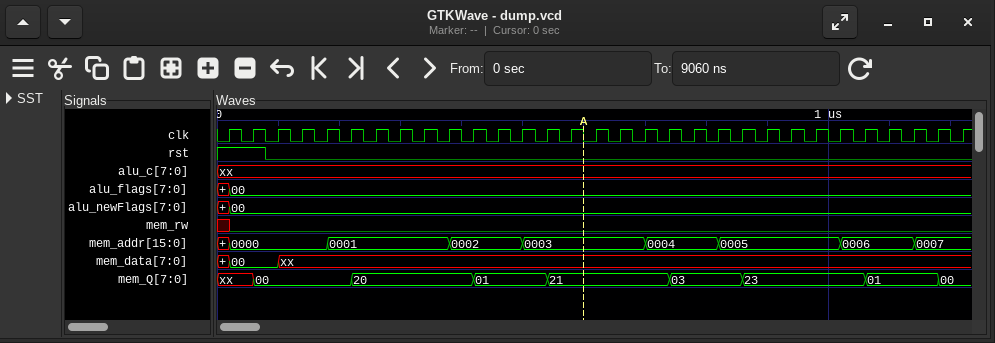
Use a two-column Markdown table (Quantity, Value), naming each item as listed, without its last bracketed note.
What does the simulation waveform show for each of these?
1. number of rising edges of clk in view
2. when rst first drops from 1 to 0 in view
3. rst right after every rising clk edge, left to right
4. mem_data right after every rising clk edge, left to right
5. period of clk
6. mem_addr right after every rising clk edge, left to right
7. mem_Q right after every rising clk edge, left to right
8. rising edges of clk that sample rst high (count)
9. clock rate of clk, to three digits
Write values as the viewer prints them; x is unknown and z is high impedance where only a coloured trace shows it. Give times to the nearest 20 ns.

| Quantity | Value |
|---|---|
| number of rising edges of clk in view | 31 |
| when rst first drops from 1 to 0 in view | 80 ns |
| rst right after every rising clk edge, left to right | 1 1 0 0 0 0 0 0 0 0 0 0 0 0 0 0 0 0 0 0 0 0 0 0 0 0 0 0 0 0 0 |
| mem_data right after every rising clk edge, left to right | 00, 00, xx, xx, xx, xx, xx, xx, xx, xx, xx, xx, xx, xx, xx, xx, xx, xx, xx, xx, xx, xx, xx, xx, xx, xx, xx, xx, xx, xx, xx |
| period of clk | 40 ns |
| mem_addr right after every rising clk edge, left to right | 0000, 0000, 0000, 0000, 0001, 0001, 0001, 0001, 0001, 0002, 0002, 0002, 0003, 0003, 0003, 0003, 0003, 0004, 0004, 0004, 0005, 0005, 0005, 0005, 0005, 0006, 0006, 0006, 0007, 0007, 0007 |
| mem_Q right after every rising clk edge, left to right | xx, 00, 00, 00, 00, 20, 20, 20, 20, 20, 01, 01, 01, 21, 21, 21, 21, 21, 03, 03, 03, 23, 23, 23, 23, 23, 01, 01, 01, 00, 00 |
| rising edges of clk that sample rst high | 2 |
| clock rate of clk, to three digits | 25.0 MHz |
